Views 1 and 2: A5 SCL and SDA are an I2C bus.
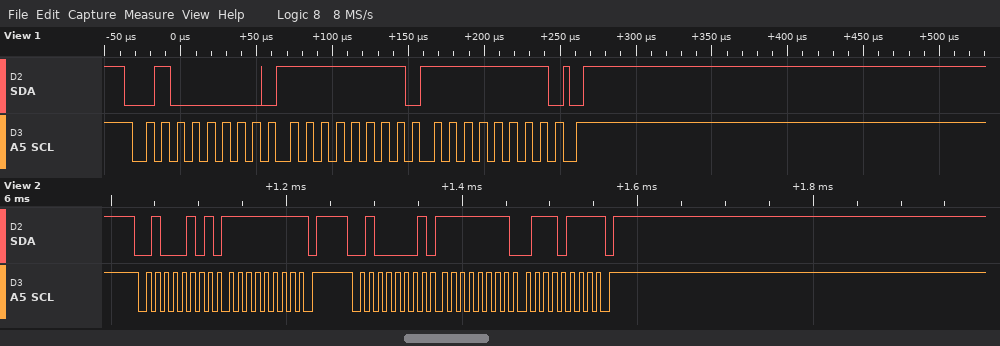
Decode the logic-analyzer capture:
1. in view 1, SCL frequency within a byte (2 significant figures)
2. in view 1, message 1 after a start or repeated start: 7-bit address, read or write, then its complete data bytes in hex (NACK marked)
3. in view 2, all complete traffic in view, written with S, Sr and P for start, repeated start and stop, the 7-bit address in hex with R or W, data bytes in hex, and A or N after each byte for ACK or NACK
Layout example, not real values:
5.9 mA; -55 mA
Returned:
100 kHz; 0x20 write: FF FF; S 22R A FF N P S 20R A FF A 77 N P
